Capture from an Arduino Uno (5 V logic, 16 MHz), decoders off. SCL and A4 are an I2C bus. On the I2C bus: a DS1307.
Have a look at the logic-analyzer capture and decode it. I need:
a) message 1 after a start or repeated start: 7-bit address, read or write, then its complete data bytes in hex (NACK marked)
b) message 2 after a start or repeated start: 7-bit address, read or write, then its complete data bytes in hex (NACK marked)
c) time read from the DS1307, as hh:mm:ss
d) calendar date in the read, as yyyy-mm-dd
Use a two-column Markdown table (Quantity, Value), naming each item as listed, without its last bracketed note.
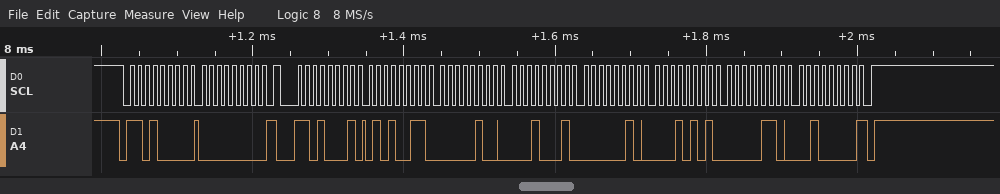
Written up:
| Quantity | Value |
|---|---|
| message 1 after a start or repeated start: 7-bit address, read or write, then its complete data bytes in hex | 0x68 write: 00 |
| message 2 after a start or repeated start: 7-bit address, read or write, then its complete data bytes in hex | 0x68 read: 53 04 11 02 15 06 20 NACK |
| time read from the DS1307, as hh:mm:ss | 11:04:53 |
| calendar date in the read, as yyyy-mm-dd | 2020-06-15 |
